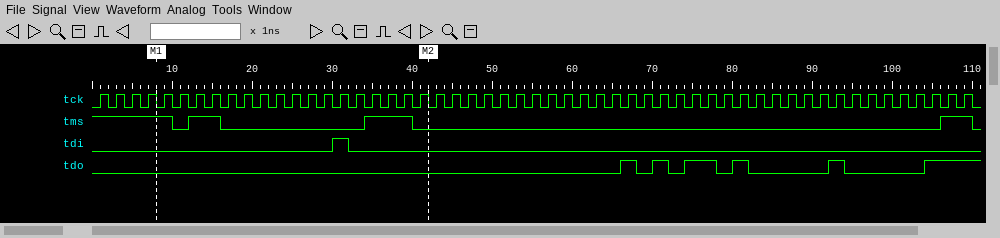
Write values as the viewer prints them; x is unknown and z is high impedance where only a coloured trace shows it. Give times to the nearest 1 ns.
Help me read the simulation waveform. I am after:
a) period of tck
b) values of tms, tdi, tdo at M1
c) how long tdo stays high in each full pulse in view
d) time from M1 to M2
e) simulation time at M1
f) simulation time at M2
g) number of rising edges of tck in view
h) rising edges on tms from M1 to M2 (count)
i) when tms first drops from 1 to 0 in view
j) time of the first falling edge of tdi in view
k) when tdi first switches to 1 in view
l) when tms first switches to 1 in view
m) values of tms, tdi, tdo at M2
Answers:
2 ns
tms=1, tdi=0, tdo=0
2 ns, 2 ns, 4 ns, 2 ns, 2 ns
34 ns
8 ns
42 ns
55
2
10 ns
32 ns
30 ns
12 ns
tms=0, tdi=0, tdo=0
